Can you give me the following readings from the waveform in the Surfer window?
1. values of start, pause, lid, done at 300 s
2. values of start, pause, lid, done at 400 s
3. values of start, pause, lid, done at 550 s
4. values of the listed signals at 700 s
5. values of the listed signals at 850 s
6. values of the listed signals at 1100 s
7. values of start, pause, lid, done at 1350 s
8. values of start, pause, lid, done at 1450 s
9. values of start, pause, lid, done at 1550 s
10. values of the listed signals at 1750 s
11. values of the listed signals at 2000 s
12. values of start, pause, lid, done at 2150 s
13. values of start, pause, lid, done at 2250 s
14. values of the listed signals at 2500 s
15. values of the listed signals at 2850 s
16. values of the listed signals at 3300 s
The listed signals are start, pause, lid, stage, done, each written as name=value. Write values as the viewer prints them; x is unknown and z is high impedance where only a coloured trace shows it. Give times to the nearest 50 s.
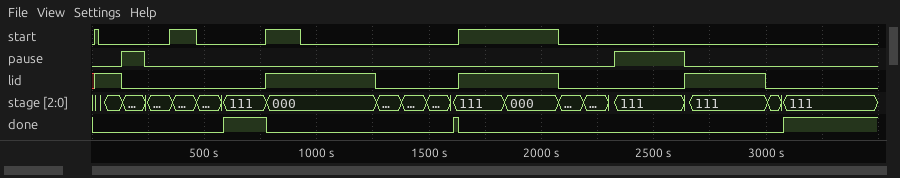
start=0, pause=0, lid=0, done=0
start=1, pause=0, lid=0, done=0
start=0, pause=0, lid=0, done=0
start=0, pause=0, lid=0, stage=111, done=1
start=1, pause=0, lid=1, stage=000, done=0
start=0, pause=0, lid=1, stage=000, done=0
start=0, pause=0, lid=0, done=0
start=0, pause=0, lid=0, done=0
start=0, pause=0, lid=0, done=0
start=1, pause=0, lid=1, stage=111, done=0
start=1, pause=0, lid=1, stage=000, done=0
start=0, pause=0, lid=0, done=0
start=0, pause=0, lid=0, done=0
start=0, pause=1, lid=0, stage=111, done=0
start=0, pause=0, lid=1, stage=111, done=0
start=0, pause=0, lid=0, stage=111, done=1
